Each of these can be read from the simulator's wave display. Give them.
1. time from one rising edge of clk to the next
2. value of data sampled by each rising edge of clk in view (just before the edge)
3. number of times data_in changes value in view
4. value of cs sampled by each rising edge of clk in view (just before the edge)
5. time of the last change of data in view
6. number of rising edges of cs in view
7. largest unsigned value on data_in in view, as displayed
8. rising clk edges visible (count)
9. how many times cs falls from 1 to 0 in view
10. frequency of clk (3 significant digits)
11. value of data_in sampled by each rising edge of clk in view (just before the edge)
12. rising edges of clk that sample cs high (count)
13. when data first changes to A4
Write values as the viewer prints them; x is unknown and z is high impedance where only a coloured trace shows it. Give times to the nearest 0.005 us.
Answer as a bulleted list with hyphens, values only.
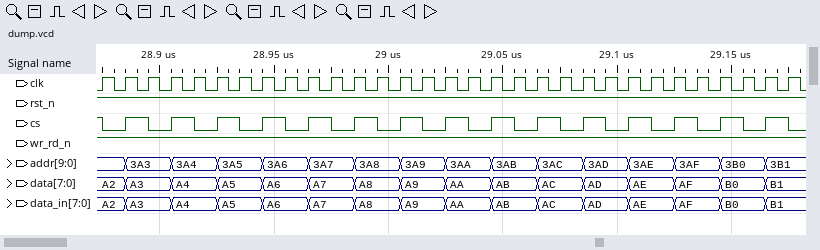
- 0.01 us
- A2, A2, A3, A3, A4, A4, A5, A5, A6, A6, A7, A7, A8, A8, A9, A9, AA, AA, AB, AB, AC, AC, AD, AD, AE, AE, AF, AF, B0, B0, B1
- 15
- 1 0 1 0 1 0 1 0 1 0 1 0 1 0 1 0 1 0 1 0 1 0 1 0 1 0 1 0 1 0 1
- 29.165 us
- 15
- B1
- 31
- 16
- 100 MHz
- A2, A2, A3, A3, A4, A4, A5, A5, A6, A6, A7, A7, A8, A8, A9, A9, AA, AA, AB, AB, AC, AC, AD, AD, AE, AE, AF, AF, B0, B0, B1
- 16
- 28.905 us
